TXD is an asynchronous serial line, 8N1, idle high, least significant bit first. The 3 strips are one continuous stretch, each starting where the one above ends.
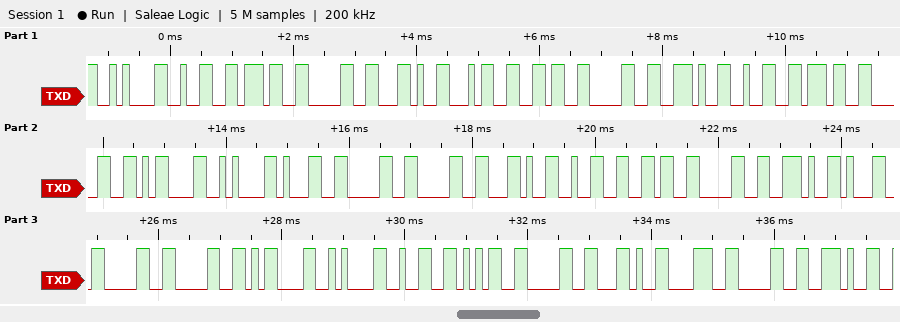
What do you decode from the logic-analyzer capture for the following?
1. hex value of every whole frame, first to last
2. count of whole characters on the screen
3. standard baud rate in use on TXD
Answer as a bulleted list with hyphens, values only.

- 0A 32 37 30 2C 34 36 30 2E 32 37 30 0D 0A 31 30 30 2C 32 36 30 2E 31 30 30 0D 0A 32 35 30 2C 38 30 2E
- 34
- 9600 baud
